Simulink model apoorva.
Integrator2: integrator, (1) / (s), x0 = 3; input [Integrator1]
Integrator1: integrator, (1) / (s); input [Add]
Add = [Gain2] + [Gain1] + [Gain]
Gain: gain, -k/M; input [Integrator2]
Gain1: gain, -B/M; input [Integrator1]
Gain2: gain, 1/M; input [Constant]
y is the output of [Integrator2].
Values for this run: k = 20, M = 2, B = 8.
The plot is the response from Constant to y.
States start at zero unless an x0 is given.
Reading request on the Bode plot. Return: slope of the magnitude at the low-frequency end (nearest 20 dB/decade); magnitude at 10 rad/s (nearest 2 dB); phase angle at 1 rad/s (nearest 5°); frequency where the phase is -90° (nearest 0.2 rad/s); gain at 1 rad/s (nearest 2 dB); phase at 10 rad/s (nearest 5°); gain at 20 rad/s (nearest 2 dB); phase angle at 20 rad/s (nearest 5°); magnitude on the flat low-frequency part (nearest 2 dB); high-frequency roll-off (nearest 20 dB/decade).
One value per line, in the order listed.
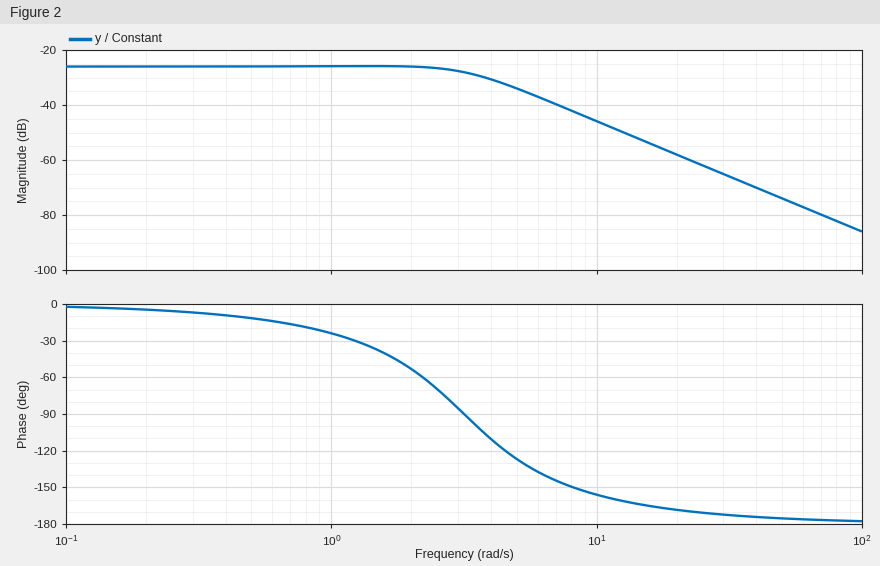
0 dB/decade
-46 dB
-25°
3.2 rad/s
-26 dB
-155°
-58 dB
-170°
-26 dB
-40 dB/decade
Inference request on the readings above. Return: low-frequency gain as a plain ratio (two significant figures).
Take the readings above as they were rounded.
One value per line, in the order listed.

0.050
